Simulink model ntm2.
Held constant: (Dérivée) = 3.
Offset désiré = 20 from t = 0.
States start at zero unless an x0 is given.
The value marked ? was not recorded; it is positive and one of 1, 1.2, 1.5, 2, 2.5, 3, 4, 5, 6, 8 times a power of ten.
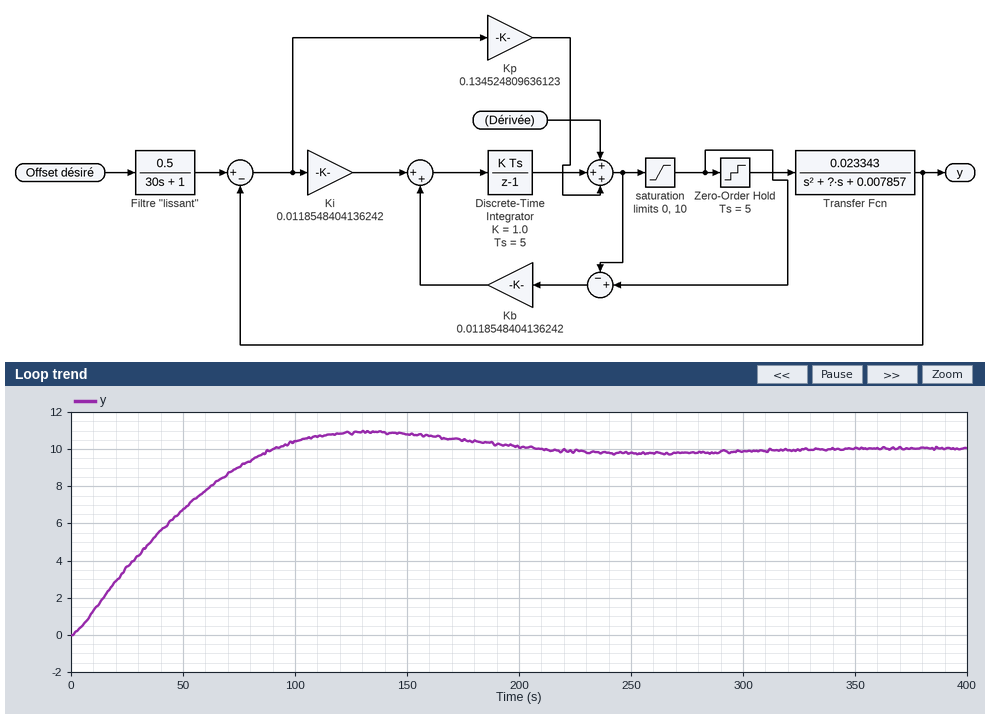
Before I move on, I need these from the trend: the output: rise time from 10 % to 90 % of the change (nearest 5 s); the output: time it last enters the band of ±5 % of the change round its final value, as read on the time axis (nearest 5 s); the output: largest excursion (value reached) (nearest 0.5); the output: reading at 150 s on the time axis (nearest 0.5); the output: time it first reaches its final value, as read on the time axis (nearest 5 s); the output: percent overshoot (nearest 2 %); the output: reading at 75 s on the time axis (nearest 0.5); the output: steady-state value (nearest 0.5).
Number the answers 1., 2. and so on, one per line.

1. 65 s
2. 175 s
3. 11.0
4. 11.0
5. 90 s
6. 10 %
7. 9.0
8. 10.0
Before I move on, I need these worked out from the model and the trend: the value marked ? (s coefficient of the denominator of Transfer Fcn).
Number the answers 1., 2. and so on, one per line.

1. 0.4
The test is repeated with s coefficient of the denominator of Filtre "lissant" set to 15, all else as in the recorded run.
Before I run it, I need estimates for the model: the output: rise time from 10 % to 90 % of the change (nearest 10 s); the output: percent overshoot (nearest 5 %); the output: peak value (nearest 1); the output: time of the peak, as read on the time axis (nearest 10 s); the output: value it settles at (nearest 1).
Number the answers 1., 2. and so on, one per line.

1. 50 s
2. 20 %
3. 12
4. 110 s
5. 10
